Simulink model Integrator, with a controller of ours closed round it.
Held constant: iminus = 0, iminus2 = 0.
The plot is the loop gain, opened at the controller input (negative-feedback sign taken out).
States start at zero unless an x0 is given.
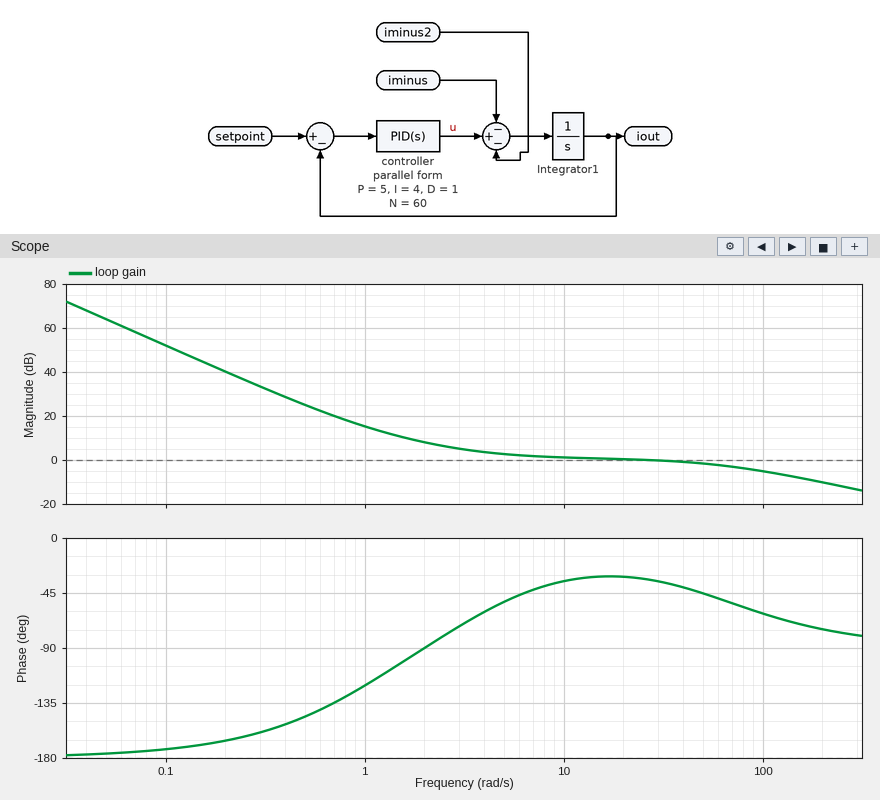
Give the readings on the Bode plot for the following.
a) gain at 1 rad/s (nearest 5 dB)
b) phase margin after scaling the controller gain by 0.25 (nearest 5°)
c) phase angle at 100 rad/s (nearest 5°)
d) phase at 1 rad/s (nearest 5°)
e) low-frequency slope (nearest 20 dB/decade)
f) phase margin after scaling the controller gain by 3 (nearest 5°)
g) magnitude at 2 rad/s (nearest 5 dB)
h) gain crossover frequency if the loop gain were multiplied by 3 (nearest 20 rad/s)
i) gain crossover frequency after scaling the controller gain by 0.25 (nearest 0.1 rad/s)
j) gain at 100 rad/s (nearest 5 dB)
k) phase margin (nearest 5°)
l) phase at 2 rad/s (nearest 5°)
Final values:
15 dB
70°
-60°
-120°
-40 dB/decade
105°
10 dB
180 rad/s
1.3 rad/s
-5 dB
145°
-90°
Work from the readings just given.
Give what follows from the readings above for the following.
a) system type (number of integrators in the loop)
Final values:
2
